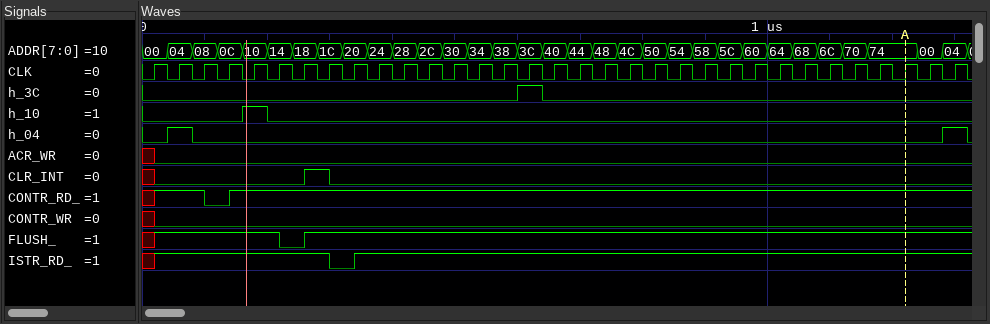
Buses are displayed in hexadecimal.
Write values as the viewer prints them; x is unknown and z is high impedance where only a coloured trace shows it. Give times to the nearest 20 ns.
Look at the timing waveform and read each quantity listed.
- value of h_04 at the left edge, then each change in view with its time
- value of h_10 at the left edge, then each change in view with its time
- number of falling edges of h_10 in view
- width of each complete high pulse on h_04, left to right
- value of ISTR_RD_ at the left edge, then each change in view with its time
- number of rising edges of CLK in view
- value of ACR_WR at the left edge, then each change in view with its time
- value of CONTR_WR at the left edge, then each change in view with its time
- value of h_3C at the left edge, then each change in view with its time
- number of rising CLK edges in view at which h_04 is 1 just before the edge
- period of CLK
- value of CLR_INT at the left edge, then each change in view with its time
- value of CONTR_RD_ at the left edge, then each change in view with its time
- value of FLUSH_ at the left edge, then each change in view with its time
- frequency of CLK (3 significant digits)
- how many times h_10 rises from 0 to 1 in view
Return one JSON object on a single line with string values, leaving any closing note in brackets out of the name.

{"value of h_04 at the left edge, then each change in view with its time": "0, 1 at 40 ns, 0 at 80 ns, 1 at 1280 ns, 0 at 1320 ns", "value of h_10 at the left edge, then each change in view with its time": "0, 1 at 160 ns, 0 at 200 ns", "number of falling edges of h_10 in view": "1", "width of each complete high pulse on h_04, left to right": "40 ns, 40 ns", "value of ISTR_RD_ at the left edge, then each change in view with its time": "x, 1 at 20 ns, 0 at 300 ns, 1 at 340 ns", "number of rising edges of CLK in view": "33", "value of ACR_WR at the left edge, then each change in view with its time": "x, 0 at 20 ns", "value of CONTR_WR at the left edge, then each change in view with its time": "x, 0 at 20 ns", "value of h_3C at the left edge, then each change in view with its time": "0, 1 at 600 ns, 0 at 640 ns", "number of rising CLK edges in view at which h_04 is 1 just before the edge": "2", "period of CLK": "40 ns", "value of CLR_INT at the left edge, then each change in view with its time": "x, 0 at 20 ns, 1 at 260 ns, 0 at 300 ns", "value of CONTR_RD_ at the left edge, then each change in view with its time": "x, 1 at 20 ns, 0 at 100 ns, 1 at 140 ns", "value of FLUSH_ at the left edge, then each change in view with its time": "x, 1 at 20 ns, 0 at 220 ns, 1 at 260 ns", "frequency of CLK": "25.0 MHz", "how many times h_10 rises from 0 to 1 in view": "1"}
